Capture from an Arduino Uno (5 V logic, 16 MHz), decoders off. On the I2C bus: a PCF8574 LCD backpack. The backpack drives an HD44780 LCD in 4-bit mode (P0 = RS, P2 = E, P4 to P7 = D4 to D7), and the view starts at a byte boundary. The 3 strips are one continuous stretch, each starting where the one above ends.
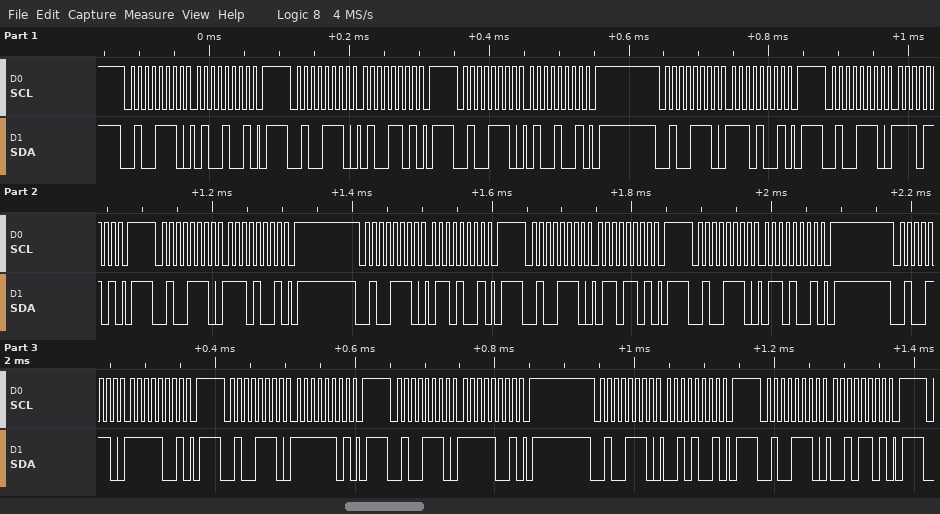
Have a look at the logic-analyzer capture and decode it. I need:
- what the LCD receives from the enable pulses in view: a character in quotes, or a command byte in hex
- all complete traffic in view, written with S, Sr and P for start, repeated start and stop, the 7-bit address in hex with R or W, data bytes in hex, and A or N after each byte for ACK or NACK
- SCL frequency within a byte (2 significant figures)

'N' 'o'
S 27W A 49 A P S 27W A 4D A P S 27W A 49 A P S 27W A E9 A P S 27W A ED A P S 27W A E9 A P S 27W A 69 A P S 27W A 6D A P S 27W A 69 A P S 27W A F9 A P S 27W A FD A P S 27W A F9 A P S 27W A 29 A P S 27W A 2D A P
100 kHz
